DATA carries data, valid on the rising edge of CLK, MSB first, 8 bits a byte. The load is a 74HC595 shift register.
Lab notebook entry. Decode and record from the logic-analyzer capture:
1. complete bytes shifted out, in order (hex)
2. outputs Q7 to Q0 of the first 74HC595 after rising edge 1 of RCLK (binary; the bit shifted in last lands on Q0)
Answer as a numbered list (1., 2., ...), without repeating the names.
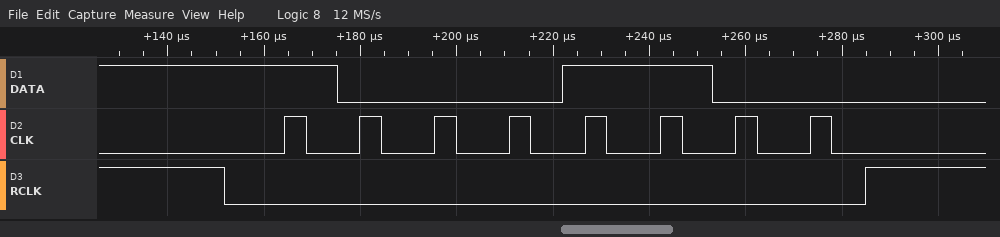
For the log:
1. 8C
2. 10001100
